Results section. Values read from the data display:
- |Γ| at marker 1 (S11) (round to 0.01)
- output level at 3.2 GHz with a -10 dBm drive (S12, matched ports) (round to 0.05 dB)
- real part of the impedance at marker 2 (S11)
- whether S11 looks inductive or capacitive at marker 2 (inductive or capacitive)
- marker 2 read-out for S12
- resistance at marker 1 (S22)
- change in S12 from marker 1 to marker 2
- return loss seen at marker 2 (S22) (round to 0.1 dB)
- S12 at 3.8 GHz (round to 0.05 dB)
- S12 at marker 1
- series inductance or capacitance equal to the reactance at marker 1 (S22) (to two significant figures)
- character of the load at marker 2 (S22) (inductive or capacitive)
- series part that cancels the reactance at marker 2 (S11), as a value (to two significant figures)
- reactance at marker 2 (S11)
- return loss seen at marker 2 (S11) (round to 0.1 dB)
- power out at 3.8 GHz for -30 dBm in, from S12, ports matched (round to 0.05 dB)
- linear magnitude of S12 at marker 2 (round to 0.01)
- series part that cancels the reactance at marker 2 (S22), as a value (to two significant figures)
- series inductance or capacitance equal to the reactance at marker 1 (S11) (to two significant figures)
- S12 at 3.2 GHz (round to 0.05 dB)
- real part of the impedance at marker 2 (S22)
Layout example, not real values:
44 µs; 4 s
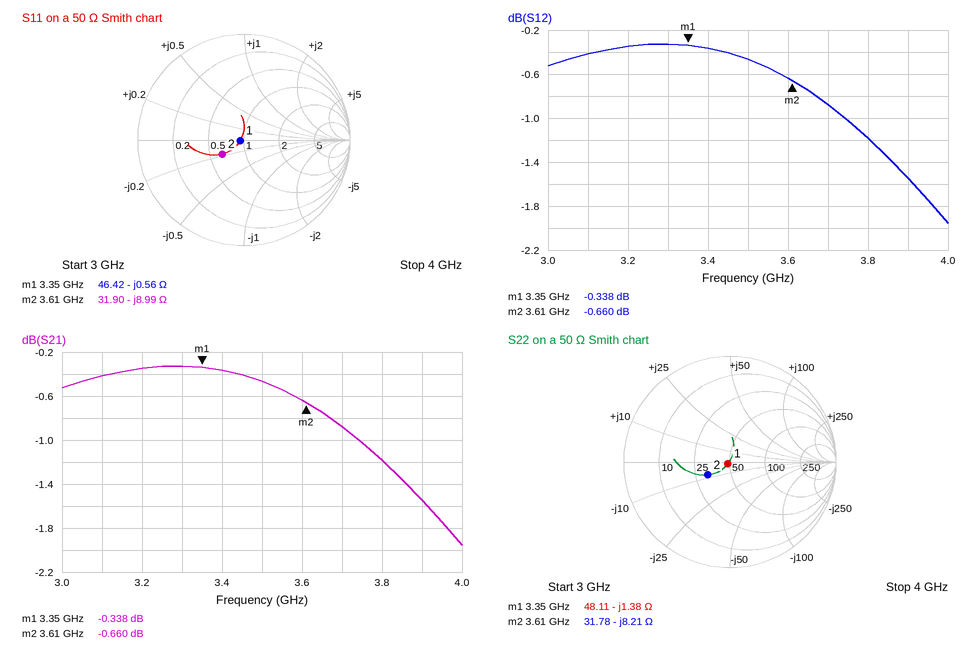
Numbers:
0.04; -10.35 dBm; 31.90 Ω; capacitive; -0.660 dB; 48.11 Ω; -0.322 dB; 12.3 dB; -1.20 dB; -0.338 dB; 34 pF; capacitive; 400 pH; -8.99 Ω; 12.2 dB; -31.20 dBm; 0.93; 360 pH; 85 pF; -0.35 dB; 31.78 Ω
